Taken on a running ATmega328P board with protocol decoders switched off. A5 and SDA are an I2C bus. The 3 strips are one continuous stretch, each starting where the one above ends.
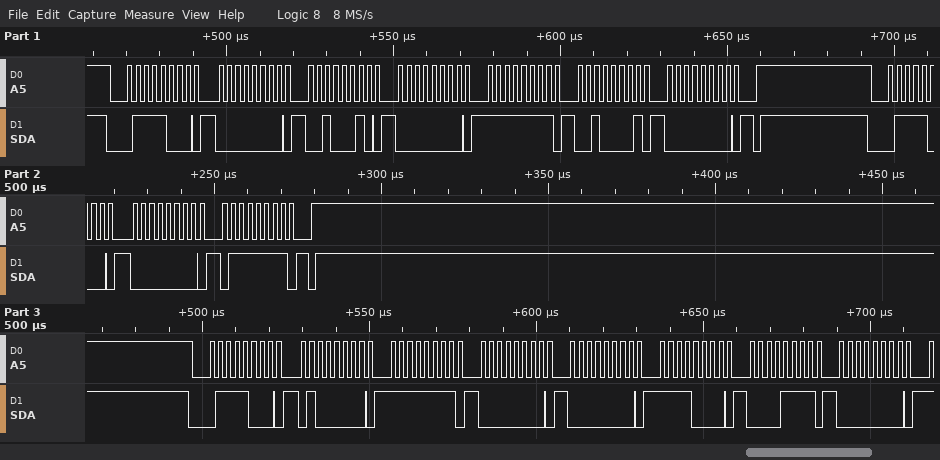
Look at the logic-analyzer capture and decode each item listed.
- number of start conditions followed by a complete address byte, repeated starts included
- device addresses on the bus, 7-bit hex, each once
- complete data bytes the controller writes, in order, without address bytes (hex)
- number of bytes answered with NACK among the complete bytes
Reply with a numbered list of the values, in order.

1. 3
2. 0x3C
3. 00 22 00 FF 21 00 00 7F 40 FF 00 00 F0 0F 00
4. 0
